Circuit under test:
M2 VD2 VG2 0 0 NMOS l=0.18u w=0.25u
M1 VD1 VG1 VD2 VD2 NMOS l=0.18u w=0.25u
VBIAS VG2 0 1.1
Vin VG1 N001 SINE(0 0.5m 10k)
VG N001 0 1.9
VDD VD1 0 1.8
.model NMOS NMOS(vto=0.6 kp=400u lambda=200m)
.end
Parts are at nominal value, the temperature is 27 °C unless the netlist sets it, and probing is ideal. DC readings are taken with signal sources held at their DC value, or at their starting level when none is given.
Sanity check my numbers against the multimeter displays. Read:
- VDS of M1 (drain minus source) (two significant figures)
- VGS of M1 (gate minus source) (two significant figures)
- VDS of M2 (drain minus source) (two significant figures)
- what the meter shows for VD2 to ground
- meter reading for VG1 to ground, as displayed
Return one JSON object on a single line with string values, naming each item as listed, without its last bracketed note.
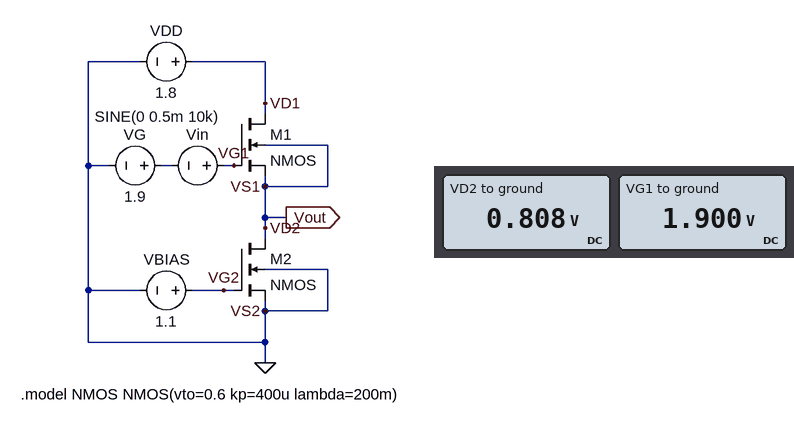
{"VDS of M1 (drain minus source)": "990 mV", "VGS of M1 (gate minus source)": "1.1 V", "VDS of M2 (drain minus source)": "810 mV", "what the meter shows for VD2 to ground": "0.808 V", "meter reading for VG1 to ground, as displayed": "1.900 V"}
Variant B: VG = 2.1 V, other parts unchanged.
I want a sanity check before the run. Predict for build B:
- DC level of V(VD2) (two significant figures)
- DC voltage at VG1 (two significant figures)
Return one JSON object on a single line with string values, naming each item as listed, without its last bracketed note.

{"DC level of V(VD2)": "990 mV", "DC voltage at VG1": "2.1 V"}
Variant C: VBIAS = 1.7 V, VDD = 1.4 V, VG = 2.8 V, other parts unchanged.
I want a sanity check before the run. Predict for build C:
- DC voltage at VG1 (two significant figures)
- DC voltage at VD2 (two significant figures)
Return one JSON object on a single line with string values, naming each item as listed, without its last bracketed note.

{"DC voltage at VG1": "2.8 V", "DC voltage at VD2": "840 mV"}
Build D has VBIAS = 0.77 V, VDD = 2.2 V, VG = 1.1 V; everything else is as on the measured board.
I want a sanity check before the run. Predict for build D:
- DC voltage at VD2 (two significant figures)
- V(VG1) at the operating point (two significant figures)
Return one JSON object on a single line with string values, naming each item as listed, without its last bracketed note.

{"DC voltage at VD2": "350 mV", "V(VG1) at the operating point": "1.1 V"}
